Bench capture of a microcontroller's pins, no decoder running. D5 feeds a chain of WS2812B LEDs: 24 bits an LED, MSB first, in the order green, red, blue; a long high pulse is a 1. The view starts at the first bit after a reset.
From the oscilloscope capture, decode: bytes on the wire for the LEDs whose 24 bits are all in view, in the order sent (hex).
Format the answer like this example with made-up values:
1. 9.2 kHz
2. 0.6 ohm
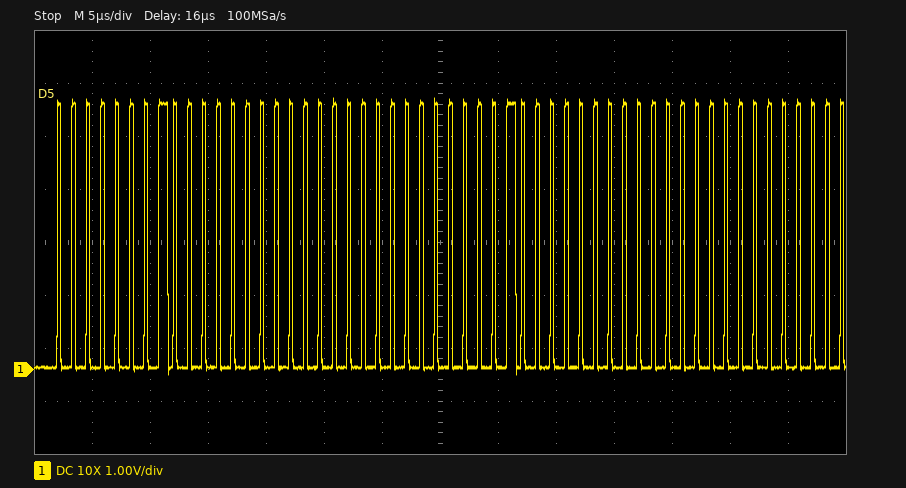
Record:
1. 01 00 00 01 00 00
